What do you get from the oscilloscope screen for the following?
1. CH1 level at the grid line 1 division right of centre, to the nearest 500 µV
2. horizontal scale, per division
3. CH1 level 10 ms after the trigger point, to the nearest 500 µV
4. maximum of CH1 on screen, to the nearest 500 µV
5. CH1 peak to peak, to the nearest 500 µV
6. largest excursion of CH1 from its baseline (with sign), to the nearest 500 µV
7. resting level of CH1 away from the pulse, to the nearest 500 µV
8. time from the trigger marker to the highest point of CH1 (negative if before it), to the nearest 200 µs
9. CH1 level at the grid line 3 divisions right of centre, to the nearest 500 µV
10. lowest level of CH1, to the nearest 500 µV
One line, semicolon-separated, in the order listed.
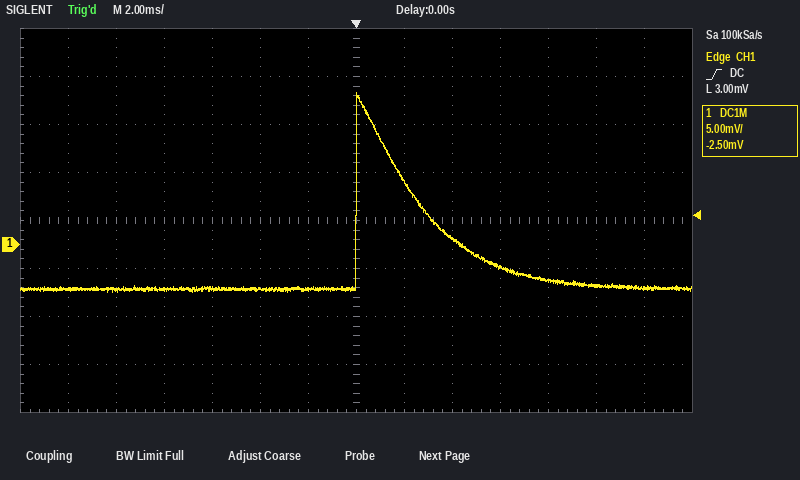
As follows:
6.5 mV; 2 ms; -4.5 mV; 16.0 mV; 21.0 mV; +20.5 mV; -4.5 mV; 0.0 ms; -2.5 mV; -5.0 mV
